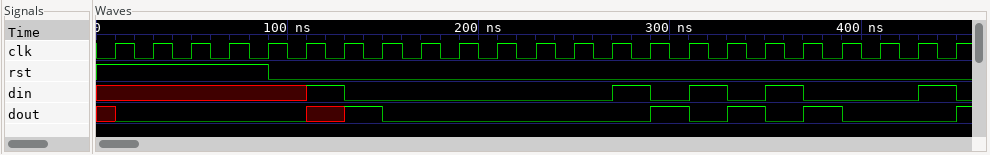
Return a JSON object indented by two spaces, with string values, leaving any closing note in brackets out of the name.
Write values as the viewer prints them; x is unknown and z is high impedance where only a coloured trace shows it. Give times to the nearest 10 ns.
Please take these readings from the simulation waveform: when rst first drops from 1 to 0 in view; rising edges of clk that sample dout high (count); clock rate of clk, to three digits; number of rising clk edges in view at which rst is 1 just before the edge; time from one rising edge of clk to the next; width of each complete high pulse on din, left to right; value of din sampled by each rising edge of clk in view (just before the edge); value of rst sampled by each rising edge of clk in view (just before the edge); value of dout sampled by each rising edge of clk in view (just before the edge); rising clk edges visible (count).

{
  "when rst first drops from 1 to 0 in view": "90 ns",
  "rising edges of clk that sample dout high": "4",
  "clock rate of clk, to three digits": "50.0 MHz",
  "number of rising clk edges in view at which rst is 1 just before the edge": "5",
  "time from one rising edge of clk to the next": "20 ns",
  "width of each complete high pulse on din, left to right": "20 ns, 20 ns, 20 ns, 20 ns",
  "value of din sampled by each rising edge of clk in view": "x x x x x x 1 0 0 0 0 0 0 0 1 0 1 0 1 0 0 0 1",
  "value of rst sampled by each rising edge of clk in view": "1 1 1 1 1 0 0 0 0 0 0 0 0 0 0 0 0 0 0 0 0 0 0",
  "value of dout sampled by each rising edge of clk in view": "x 0 0 0 0 0 x 1 0 0 0 0 0 0 0 1 0 1 0 1 0 0 0",
  "rising clk edges visible": "23"
}
